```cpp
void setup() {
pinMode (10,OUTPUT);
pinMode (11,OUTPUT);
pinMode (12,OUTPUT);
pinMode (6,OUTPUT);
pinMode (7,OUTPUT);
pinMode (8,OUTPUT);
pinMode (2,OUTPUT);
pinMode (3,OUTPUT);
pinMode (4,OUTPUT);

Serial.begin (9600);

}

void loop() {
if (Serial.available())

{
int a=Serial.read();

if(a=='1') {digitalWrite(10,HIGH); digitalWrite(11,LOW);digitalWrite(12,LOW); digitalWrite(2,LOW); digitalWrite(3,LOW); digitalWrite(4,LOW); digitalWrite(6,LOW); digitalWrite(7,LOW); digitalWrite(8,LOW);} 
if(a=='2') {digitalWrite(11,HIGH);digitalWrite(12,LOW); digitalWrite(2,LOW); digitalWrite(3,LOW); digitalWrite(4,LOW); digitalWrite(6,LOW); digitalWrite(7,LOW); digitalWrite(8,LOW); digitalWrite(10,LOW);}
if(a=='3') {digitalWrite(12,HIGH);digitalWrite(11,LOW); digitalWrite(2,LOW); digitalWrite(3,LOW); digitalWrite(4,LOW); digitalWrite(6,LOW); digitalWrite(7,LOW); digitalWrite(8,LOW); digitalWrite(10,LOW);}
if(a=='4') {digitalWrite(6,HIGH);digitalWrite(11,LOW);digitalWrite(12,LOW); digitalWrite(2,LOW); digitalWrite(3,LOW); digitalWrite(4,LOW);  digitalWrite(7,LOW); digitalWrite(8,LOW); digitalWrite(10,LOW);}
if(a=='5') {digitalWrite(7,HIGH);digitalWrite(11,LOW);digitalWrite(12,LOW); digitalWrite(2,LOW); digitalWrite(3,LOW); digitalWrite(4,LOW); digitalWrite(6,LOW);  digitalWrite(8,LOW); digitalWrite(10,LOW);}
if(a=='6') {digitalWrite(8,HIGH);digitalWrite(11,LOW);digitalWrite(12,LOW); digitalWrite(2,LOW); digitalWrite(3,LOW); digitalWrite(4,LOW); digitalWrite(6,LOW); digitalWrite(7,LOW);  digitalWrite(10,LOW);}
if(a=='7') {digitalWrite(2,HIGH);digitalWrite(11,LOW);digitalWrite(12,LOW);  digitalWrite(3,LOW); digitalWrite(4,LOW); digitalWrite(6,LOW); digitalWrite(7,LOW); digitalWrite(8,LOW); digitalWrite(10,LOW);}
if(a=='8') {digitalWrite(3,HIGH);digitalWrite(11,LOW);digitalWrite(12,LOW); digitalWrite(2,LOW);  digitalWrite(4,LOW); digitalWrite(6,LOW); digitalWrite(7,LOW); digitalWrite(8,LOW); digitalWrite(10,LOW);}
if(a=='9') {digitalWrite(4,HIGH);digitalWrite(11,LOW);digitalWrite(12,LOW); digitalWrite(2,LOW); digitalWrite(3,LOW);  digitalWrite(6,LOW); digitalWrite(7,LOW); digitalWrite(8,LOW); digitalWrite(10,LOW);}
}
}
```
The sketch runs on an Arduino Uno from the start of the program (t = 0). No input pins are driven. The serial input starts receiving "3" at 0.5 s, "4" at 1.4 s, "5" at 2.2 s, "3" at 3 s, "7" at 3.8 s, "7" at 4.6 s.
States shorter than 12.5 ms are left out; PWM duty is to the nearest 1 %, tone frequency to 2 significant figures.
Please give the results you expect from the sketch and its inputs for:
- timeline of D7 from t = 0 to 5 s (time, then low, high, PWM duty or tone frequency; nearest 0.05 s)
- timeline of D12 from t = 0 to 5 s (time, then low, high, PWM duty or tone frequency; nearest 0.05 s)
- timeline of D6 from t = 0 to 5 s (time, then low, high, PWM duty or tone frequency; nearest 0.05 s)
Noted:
0 s low; 2.2 s high; 3 s low
0 s low; 0.5 s high; 1.4 s low; 3 s high; 3.8 s low
0 s low; 1.4 s high; 2.2 s low
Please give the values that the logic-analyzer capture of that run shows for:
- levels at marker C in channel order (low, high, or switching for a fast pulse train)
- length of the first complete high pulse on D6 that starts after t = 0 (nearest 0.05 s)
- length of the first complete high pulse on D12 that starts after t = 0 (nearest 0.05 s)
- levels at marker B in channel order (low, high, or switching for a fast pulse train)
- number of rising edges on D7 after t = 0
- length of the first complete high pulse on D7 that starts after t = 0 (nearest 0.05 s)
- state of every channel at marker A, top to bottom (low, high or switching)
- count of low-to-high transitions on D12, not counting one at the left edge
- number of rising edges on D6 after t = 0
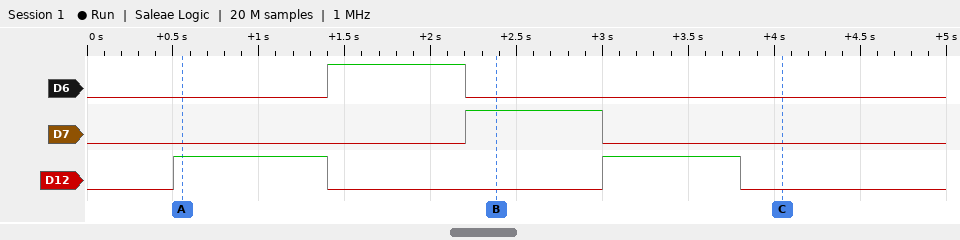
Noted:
D6 low, D7 low, D12 low
0.80 s
0.90 s
D6 low, D7 high, D12 low
1
0.80 s
D6 low, D7 low, D12 high
2
1
